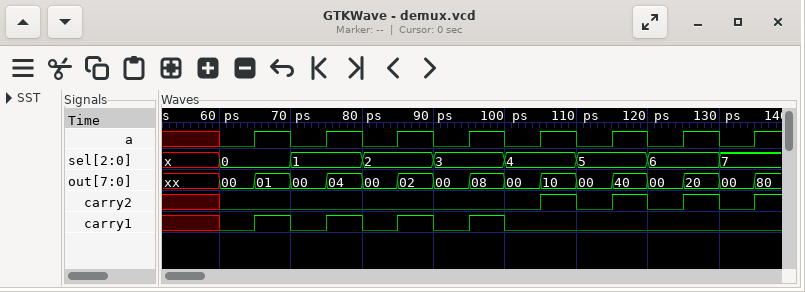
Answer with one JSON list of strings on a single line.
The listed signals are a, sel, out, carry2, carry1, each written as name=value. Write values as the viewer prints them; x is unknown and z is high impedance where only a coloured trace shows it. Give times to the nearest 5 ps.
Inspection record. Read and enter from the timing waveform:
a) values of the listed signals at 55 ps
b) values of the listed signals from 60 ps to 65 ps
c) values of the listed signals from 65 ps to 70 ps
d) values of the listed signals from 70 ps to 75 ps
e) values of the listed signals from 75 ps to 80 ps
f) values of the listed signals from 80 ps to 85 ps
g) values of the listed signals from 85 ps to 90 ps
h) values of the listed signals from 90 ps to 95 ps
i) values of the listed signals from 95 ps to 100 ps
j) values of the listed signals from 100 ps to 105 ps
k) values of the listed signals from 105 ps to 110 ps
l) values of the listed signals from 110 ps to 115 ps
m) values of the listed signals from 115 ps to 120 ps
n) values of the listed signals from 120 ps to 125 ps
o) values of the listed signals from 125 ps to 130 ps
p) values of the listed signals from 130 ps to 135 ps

["a=x, sel=x, out=xx, carry2=x, carry1=x", "a=0, sel=0, out=00, carry2=0, carry1=0", "a=1, sel=0, out=01, carry2=0, carry1=1", "a=0, sel=1, out=00, carry2=0, carry1=0", "a=1, sel=1, out=04, carry2=0, carry1=1", "a=0, sel=2, out=00, carry2=0, carry1=0", "a=1, sel=2, out=02, carry2=0, carry1=1", "a=0, sel=3, out=00, carry2=0, carry1=0", "a=1, sel=3, out=08, carry2=0, carry1=1", "a=0, sel=4, out=00, carry2=0, carry1=0", "a=1, sel=4, out=10, carry2=1, carry1=0", "a=0, sel=5, out=00, carry2=0, carry1=0", "a=1, sel=5, out=40, carry2=1, carry1=0", "a=0, sel=6, out=00, carry2=0, carry1=0", "a=1, sel=6, out=20, carry2=1, carry1=0", "a=0, sel=7, out=00, carry2=0, carry1=0"]
